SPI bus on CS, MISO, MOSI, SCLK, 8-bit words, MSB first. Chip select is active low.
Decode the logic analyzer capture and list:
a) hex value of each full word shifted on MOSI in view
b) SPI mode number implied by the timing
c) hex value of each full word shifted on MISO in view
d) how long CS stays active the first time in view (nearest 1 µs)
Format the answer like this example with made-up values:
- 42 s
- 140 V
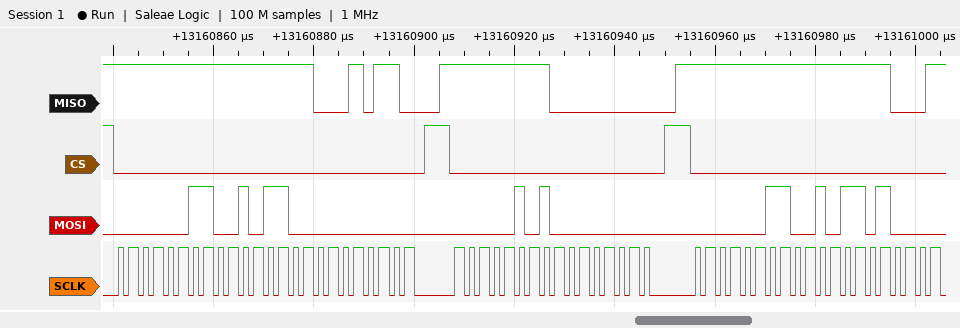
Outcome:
- 03, 2C, 00, 05, 00, 03, 2D
- 0
- FF, FF, 16, FF, 00, FF, FF
- 62 µs
